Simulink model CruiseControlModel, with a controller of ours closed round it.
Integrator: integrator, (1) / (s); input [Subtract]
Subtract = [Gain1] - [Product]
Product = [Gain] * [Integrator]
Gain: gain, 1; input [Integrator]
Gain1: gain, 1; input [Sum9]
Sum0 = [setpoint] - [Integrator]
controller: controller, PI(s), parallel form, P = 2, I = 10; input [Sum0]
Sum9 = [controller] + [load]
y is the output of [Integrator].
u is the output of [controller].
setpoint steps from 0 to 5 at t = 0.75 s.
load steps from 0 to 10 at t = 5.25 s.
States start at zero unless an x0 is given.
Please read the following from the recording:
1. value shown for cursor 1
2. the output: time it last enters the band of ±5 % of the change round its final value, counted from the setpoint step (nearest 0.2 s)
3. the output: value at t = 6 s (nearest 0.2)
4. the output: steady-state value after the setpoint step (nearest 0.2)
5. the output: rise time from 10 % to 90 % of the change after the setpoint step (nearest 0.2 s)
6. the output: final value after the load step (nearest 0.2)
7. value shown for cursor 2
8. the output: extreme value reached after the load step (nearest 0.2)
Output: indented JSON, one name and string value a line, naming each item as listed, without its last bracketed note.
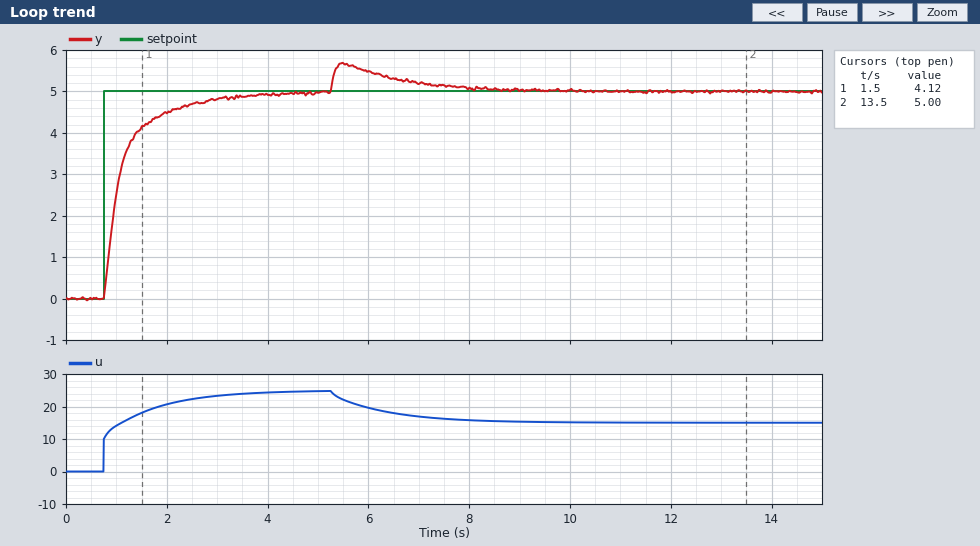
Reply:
{
  "value shown for cursor 1": "4.12",
  "the output: time it last enters the band of ±5 % of the change round its final value, counted from the setpoint step": "2.0 s",
  "the output: value at t = 6 s": "5.4",
  "the output: steady-state value after the setpoint step": "5.0",
  "the output: rise time from 10 % to 90 % of the change after the setpoint step": "1.2 s",
  "the output: final value after the load step": "5.0",
  "value shown for cursor 2": "5.00",
  "the output: extreme value reached after the load step": "5.6"
}
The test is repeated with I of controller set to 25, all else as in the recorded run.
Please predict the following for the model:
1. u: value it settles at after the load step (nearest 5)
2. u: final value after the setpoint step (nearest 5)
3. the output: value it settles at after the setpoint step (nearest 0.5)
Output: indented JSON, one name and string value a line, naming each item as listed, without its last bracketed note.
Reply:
{
  "u: value it settles at after the load step": "15",
  "u: final value after the setpoint step": "25",
  "the output: value it settles at after the setpoint step": "5.0"
}
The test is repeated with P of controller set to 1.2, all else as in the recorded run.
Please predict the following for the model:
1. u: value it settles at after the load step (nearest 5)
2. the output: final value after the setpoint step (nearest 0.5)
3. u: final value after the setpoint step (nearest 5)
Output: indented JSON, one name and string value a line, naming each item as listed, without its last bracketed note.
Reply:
{
  "u: value it settles at after the load step": "15",
  "the output: final value after the setpoint step": "5.0",
  "u: final value after the setpoint step": "25"
}
